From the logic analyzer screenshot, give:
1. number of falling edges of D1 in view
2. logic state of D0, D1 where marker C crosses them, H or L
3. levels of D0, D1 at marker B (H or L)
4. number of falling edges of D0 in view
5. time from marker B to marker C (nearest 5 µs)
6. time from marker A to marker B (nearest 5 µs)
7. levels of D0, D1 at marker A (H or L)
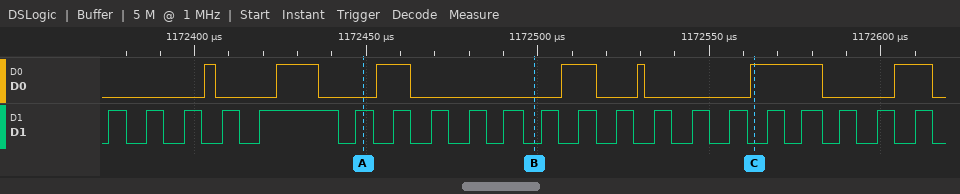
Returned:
21
D0=H, D1=L
D0=L, D1=L
7
65 µs
50 µs
D0=L, D1=H
